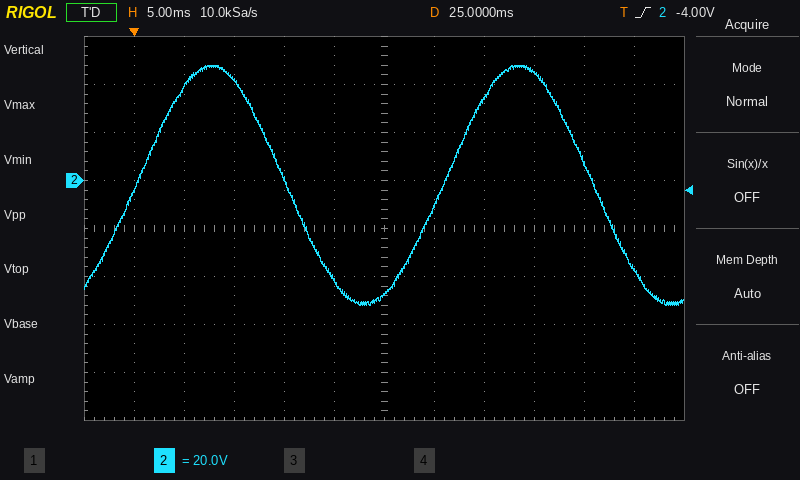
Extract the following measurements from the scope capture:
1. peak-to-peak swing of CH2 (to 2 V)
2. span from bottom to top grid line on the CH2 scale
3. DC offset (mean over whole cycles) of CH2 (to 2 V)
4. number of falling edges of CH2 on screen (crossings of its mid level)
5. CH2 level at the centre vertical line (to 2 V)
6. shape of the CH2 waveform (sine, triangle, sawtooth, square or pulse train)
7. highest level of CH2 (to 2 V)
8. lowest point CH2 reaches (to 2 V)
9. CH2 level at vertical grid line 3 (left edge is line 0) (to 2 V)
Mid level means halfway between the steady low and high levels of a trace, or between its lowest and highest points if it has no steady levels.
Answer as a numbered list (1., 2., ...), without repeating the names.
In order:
1. 100 V
2. 160 V
3. -2 V
4. 2
5. -48 V
6. sine
7. 48 V
8. -52 V
9. 42 V
